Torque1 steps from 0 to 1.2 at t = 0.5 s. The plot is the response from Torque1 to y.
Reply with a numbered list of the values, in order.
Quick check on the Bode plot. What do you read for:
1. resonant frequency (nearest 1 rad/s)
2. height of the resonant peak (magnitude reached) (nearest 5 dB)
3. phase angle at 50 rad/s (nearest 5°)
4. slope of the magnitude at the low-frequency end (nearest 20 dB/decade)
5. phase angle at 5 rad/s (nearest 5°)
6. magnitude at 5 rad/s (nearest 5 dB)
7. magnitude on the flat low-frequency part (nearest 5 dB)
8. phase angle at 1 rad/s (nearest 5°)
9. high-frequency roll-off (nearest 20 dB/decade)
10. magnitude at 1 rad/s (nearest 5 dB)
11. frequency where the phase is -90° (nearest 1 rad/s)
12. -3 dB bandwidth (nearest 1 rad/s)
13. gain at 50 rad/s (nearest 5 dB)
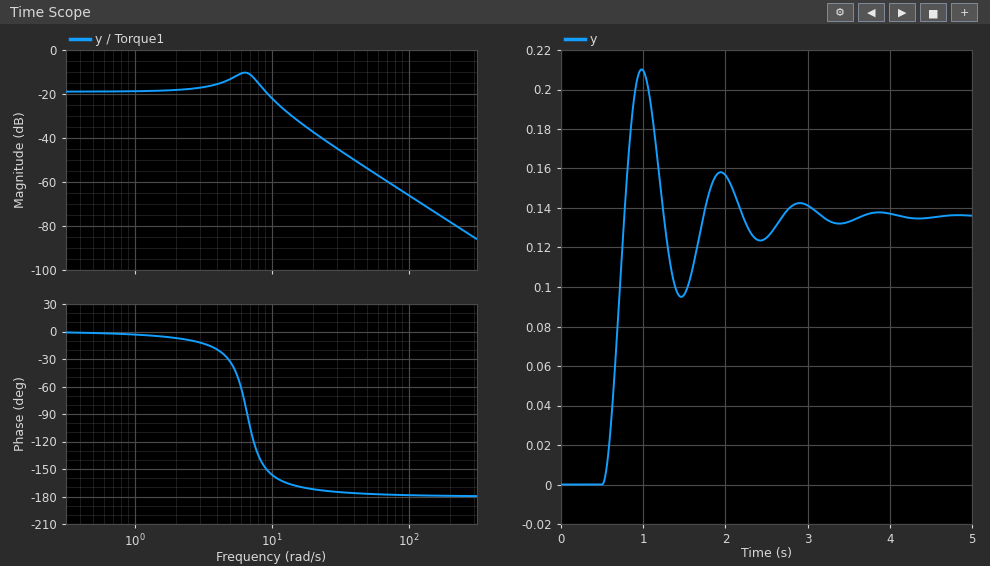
1. 6 rad/s
2. -10 dB
3. -175°
4. 0 dB/decade
5. -35°
6. -15 dB
7. -20 dB
8. -5°
9. -40 dB/decade
10. -20 dB
11. 7 rad/s
12. 10 rad/s
13. -55 dB
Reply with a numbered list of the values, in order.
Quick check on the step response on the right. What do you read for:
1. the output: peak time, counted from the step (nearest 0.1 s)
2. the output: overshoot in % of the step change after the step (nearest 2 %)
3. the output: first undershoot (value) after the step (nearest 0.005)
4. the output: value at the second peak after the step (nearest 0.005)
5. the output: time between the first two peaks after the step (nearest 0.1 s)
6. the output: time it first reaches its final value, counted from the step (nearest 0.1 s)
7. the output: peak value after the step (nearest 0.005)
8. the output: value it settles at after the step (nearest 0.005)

1. 0.5 s
2. 54 %
3. 0.095
4. 0.160
5. 1.0 s
6. 0.3 s
7. 0.210
8. 0.135
